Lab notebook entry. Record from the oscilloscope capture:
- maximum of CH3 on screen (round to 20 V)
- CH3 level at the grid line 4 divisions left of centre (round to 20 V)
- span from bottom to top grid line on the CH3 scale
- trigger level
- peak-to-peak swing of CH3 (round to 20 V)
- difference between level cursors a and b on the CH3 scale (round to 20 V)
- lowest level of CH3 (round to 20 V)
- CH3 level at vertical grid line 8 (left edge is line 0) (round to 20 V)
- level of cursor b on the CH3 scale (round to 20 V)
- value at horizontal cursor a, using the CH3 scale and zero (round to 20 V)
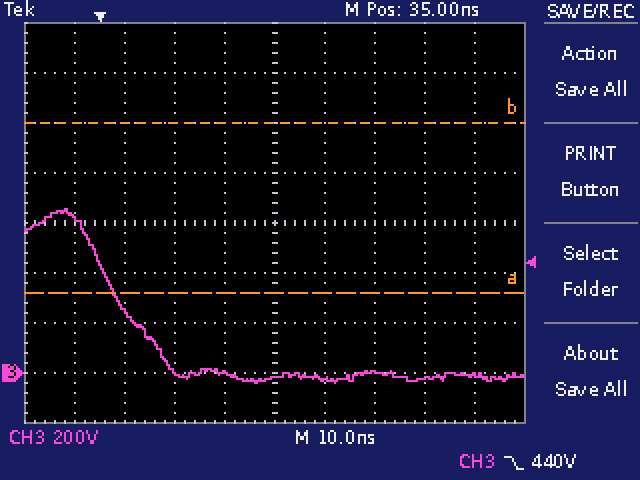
660 V
620 V
1.6 kV
440 V
700 V
680 V
-40 V
-20 V
1.00 kV
320 V
